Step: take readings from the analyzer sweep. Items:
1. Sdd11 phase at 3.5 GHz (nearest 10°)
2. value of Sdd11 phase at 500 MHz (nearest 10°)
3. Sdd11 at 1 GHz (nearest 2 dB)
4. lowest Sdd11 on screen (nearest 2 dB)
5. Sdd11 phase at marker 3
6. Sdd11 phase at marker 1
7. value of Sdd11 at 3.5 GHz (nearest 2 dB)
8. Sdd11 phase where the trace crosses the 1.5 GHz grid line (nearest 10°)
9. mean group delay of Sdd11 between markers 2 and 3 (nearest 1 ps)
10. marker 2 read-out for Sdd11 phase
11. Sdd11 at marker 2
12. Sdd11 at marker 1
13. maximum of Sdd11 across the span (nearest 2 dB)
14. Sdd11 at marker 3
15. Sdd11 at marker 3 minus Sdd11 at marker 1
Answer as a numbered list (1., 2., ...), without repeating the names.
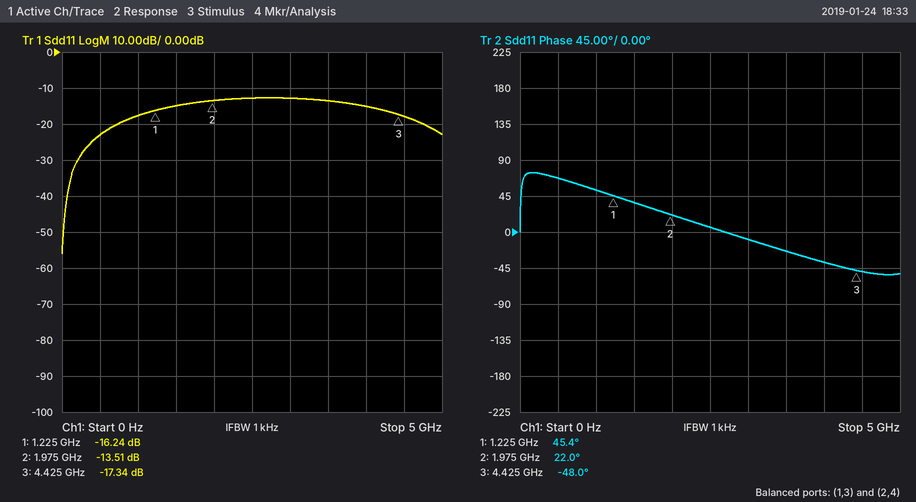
1. -20°
2. 70°
3. -18 dB
4. -56 dB
5. -48.0°
6. 45.4°
7. -14 dB
8. 40°
9. 79 ps
10. 22.0°
11. -13.51 dB
12. -16.24 dB
13. -12 dB
14. -17.34 dB
15. -1.10 dB
